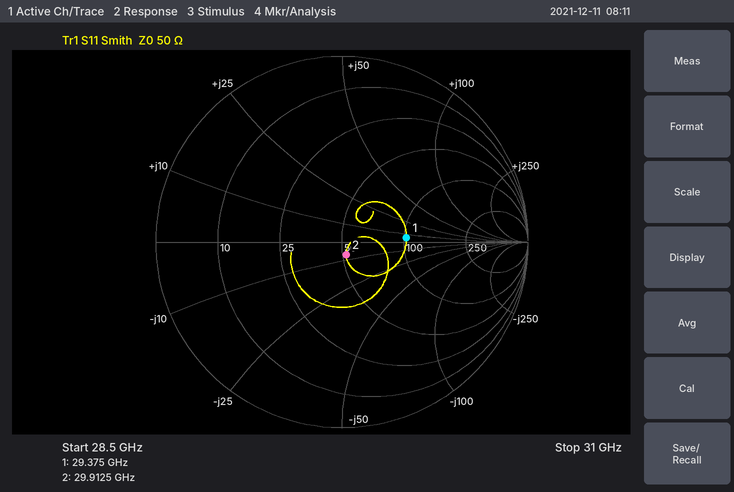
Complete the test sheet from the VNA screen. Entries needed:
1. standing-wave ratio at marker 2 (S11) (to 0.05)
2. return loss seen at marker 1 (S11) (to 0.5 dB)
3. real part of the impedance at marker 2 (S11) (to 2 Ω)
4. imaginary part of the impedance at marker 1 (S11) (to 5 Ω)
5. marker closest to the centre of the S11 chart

1.15
9.0 dB
52 Ω
+5 Ω
marker 2
